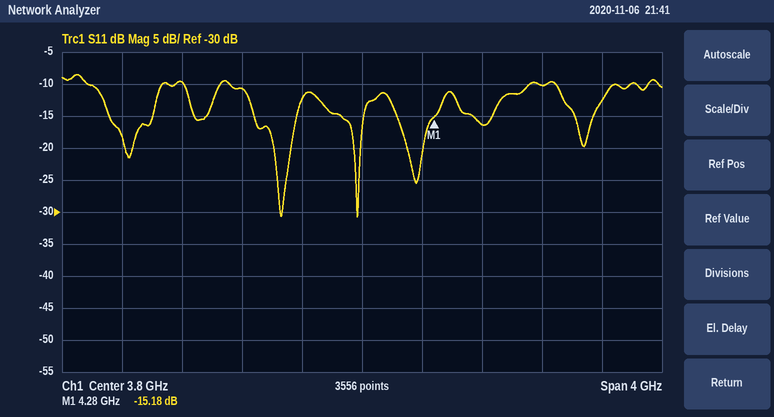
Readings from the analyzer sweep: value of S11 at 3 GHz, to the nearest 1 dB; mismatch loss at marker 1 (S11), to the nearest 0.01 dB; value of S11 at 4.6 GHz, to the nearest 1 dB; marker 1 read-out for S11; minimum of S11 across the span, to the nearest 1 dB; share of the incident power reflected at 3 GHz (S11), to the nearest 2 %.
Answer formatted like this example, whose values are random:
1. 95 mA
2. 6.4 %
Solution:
1. -11 dB
2. 0.13 dB
3. -16 dB
4. -15.18 dB
5. -31 dB
6. 8 %
